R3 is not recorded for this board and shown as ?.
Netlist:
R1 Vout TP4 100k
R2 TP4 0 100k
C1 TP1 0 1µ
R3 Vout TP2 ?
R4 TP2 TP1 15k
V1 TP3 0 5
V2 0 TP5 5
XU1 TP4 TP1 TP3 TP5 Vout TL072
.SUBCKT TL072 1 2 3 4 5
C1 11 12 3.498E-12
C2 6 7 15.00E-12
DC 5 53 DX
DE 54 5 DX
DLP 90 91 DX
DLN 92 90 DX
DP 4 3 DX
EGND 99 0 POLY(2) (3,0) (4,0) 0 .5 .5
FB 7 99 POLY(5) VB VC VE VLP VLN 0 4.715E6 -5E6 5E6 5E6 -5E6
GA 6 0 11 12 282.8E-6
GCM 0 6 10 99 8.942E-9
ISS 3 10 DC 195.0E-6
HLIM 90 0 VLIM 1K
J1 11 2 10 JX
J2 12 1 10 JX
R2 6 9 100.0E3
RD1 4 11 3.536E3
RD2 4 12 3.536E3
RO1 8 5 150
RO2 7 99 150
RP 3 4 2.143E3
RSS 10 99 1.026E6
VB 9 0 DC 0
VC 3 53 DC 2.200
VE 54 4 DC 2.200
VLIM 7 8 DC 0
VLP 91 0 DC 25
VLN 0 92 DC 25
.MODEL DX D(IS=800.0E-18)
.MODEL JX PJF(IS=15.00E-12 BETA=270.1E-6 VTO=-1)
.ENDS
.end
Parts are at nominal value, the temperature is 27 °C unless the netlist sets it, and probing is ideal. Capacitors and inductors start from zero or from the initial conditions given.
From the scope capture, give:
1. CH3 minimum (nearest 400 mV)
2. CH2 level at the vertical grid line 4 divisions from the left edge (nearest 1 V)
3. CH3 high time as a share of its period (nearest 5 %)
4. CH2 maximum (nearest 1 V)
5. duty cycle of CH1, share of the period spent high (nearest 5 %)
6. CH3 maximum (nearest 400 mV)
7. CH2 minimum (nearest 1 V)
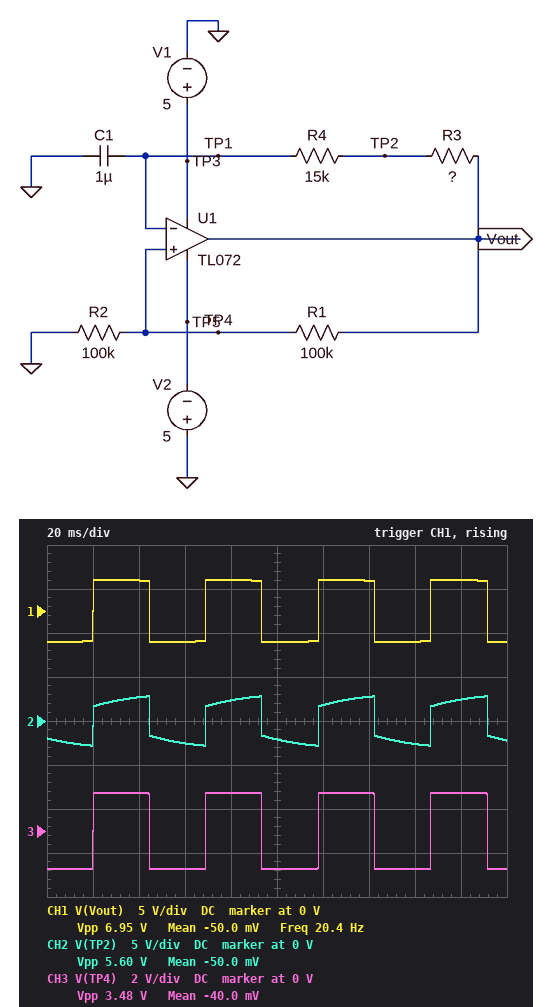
-1.6 V
2 V
50 %
3 V
50 %
1.6 V
-3 V
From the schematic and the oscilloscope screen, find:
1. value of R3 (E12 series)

8.2 kΩ
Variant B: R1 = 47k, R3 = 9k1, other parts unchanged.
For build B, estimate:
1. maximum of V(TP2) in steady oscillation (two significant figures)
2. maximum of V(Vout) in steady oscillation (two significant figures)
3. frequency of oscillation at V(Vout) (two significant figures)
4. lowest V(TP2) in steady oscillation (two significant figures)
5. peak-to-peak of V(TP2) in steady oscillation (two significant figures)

3.0 V
3.5 V
13 Hz
-3.0 V
6.0 V
